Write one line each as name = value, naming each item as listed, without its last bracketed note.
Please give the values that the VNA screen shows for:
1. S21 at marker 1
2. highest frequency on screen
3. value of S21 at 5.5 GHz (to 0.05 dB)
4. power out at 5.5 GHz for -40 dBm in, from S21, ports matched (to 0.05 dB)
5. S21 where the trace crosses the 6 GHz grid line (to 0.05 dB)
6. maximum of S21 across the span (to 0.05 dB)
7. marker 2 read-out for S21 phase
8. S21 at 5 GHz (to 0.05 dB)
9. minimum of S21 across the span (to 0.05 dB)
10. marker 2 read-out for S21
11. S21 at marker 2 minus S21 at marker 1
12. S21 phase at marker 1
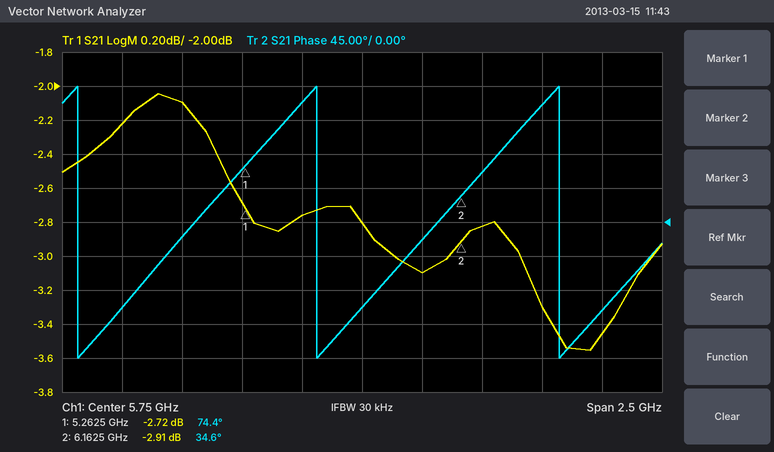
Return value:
S21 at marker 1 = -2.72 dB
highest frequency on screen = 7 GHz
value of S21 at 5.5 GHz = -2.75 dB
power out at 5.5 GHz for -40 dBm in, from S21, ports matched = -42.75 dBm
S21 where the trace crosses the 6 GHz grid line = -3.10 dB
maximum of S21 across the span = -2.05 dB
marker 2 read-out for S21 phase = 34.6°
S21 at 5 GHz = -2.10 dB
minimum of S21 across the span = -3.55 dB
marker 2 read-out for S21 = -2.91 dB
S21 at marker 2 minus S21 at marker 1 = -0.19 dB
S21 phase at marker 1 = 74.4°
